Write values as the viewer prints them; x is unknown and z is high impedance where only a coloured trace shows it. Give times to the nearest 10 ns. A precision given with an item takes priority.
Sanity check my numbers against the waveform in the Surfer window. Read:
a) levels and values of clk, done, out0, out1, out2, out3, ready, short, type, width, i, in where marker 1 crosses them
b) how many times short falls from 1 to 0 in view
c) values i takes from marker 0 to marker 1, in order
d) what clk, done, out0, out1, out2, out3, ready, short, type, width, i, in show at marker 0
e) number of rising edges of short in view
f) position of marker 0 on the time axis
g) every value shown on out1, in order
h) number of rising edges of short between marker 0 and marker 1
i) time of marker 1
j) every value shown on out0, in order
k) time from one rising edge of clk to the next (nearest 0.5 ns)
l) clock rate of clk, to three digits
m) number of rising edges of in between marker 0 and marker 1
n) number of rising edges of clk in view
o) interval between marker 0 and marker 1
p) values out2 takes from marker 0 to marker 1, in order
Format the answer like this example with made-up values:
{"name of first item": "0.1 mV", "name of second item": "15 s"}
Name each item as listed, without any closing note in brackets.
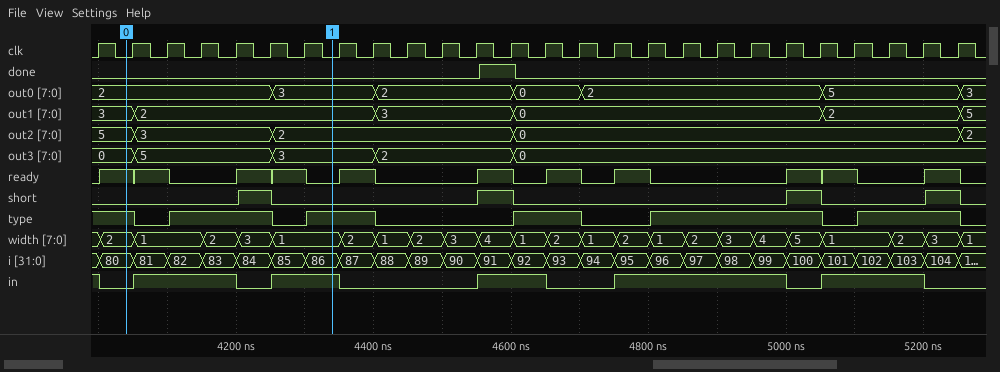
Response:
{"levels and values of clk, done, out0, out1, out2, out3, ready, short, type, width, i, in where marker 1 crosses them": "clk=0, done=0, out0=3, out1=2, out2=2, out3=3, ready=0, short=0, type=1, width=1, i=86, in=1", "how many times short falls from 1 to 0 in view": "4", "values i takes from marker 0 to marker 1, in order": "80, 81, 82, 83, 84, 85, 86", "what clk, done, out0, out1, out2, out3, ready, short, type, width, i, in show at marker 0": "clk=0, done=0, out0=2, out1=3, out2=5, out3=0, ready=1, short=0, type=1, width=2, i=80, in=0", "number of rising edges of short in view": "4", "position of marker 0 on the time axis": "4040 ns", "every value shown on out1, in order": "3, 2, 3, 0, 2, 5", "number of rising edges of short between marker 0 and marker 1": "1", "time of marker 1": "4340 ns", "every value shown on out0, in order": "2, 3, 2, 0, 2, 5, 3", "time from one rising edge of clk to the next": "50 ns", "clock rate of clk, to three digits": "20.0 MHz", "number of rising edges of in between marker 0 and marker 1": "2", "number of rising edges of clk in view": "26", "interval between marker 0 and marker 1": "300 ns", "values out2 takes from marker 0 to marker 1, in order": "5, 3, 2"}
